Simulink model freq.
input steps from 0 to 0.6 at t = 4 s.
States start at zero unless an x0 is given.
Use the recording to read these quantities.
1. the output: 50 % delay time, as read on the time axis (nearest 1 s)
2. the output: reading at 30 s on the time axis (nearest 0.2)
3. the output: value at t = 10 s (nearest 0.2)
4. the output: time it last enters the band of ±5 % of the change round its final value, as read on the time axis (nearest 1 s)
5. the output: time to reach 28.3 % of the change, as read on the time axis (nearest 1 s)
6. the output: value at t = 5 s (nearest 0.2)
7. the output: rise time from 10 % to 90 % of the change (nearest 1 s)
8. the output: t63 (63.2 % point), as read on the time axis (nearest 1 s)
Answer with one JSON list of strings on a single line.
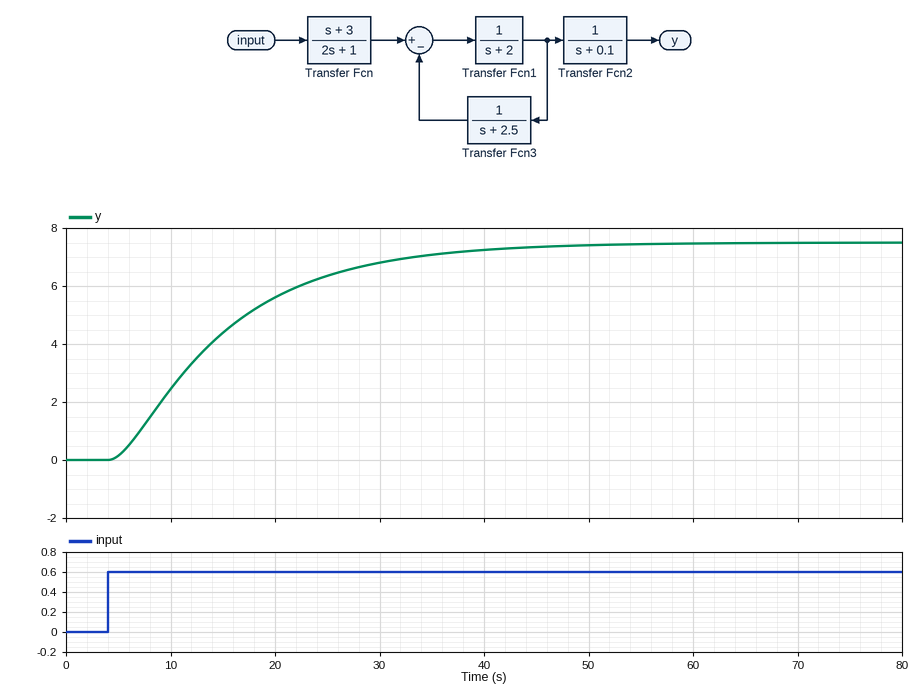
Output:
["13 s", "6.8", "2.4", "36 s", "9 s", "0.2", "23 s", "16 s"]
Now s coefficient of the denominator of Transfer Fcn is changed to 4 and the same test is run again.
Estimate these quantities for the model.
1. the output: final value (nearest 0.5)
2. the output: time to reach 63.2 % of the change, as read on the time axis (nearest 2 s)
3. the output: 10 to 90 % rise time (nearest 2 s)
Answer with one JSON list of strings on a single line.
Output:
["7.5", "18 s", "24 s"]
